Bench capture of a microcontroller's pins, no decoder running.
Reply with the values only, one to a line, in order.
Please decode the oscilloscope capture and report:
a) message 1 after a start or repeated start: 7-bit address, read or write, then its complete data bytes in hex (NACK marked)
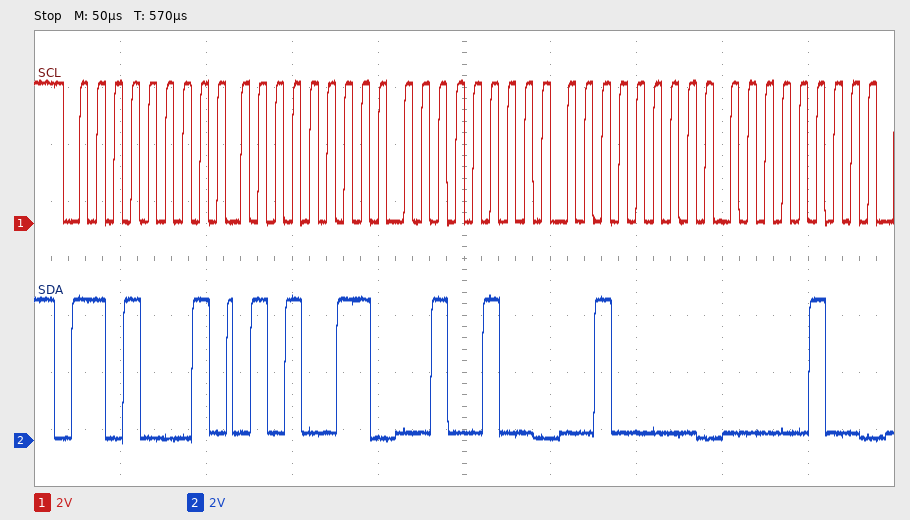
0x68 read: 53 24 20 04
